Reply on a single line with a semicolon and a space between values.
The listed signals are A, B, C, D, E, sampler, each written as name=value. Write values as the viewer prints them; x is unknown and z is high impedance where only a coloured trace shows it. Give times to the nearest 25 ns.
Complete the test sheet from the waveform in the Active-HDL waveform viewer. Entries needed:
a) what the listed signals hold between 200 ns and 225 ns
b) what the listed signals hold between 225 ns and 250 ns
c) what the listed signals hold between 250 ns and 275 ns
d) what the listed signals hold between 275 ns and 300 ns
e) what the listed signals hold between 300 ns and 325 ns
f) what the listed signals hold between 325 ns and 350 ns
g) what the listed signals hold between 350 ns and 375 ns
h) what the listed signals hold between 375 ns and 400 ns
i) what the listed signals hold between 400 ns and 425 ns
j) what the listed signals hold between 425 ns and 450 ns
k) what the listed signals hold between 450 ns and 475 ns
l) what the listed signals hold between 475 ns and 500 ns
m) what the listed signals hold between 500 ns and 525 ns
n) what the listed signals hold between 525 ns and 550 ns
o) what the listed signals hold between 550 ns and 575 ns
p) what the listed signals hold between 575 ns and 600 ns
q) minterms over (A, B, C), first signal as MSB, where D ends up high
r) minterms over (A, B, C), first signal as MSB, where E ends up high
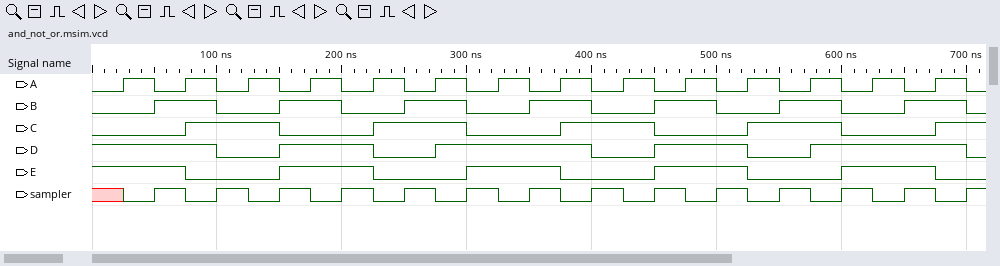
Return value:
A=0, B=0, C=0, D=1, E=1, sampler=1; A=1, B=0, C=1, D=0, E=0, sampler=0; A=0, B=1, C=1, D=0, E=0, sampler=1; A=1, B=1, C=1, D=1, E=0, sampler=0; A=0, B=0, C=0, D=1, E=1, sampler=1; A=1, B=0, C=0, D=1, E=1, sampler=0; A=0, B=1, C=0, D=1, E=1, sampler=1; A=1, B=1, C=1, D=1, E=0, sampler=0; A=0, B=0, C=1, D=0, E=0, sampler=1; A=1, B=0, C=1, D=0, E=0, sampler=0; A=0, B=1, C=0, D=1, E=1, sampler=1; A=1, B=1, C=0, D=1, E=1, sampler=0; A=0, B=0, C=0, D=1, E=1, sampler=1; A=1, B=0, C=1, D=0, E=0, sampler=0; A=0, B=1, C=1, D=0, E=0, sampler=1; A=1, B=1, C=1, D=1, E=0, sampler=0; 0, 2, 4, 6, 7; 0, 2, 4, 6
